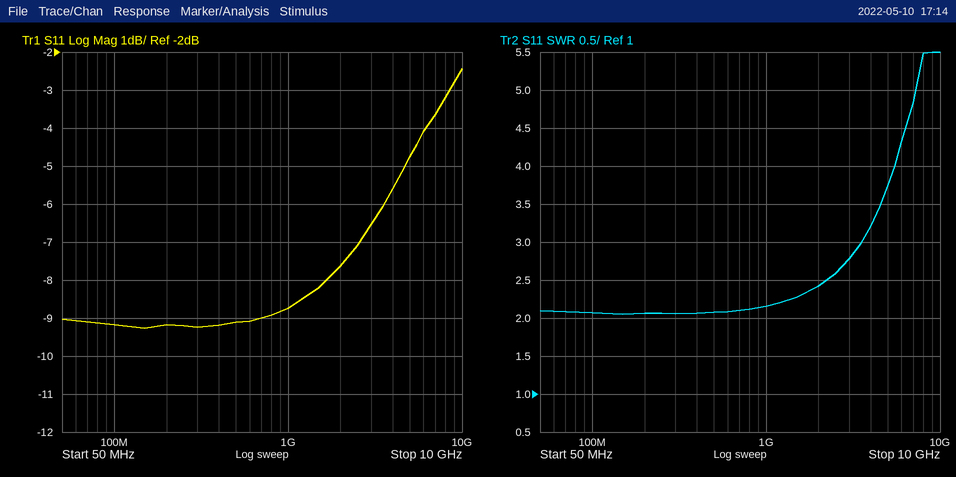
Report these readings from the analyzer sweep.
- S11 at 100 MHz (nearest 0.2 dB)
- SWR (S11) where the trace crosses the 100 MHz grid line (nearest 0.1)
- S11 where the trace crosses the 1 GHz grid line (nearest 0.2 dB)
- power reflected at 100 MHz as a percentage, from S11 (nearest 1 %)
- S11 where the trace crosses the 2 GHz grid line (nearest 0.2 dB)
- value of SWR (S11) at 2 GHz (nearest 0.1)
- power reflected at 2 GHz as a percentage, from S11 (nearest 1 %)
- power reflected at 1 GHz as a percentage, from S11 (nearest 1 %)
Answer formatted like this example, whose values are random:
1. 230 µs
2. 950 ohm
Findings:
1. -9.2 dB
2. 2.1
3. -8.8 dB
4. 12 %
5. -7.6 dB
6. 2.4
7. 17 %
8. 13 %
